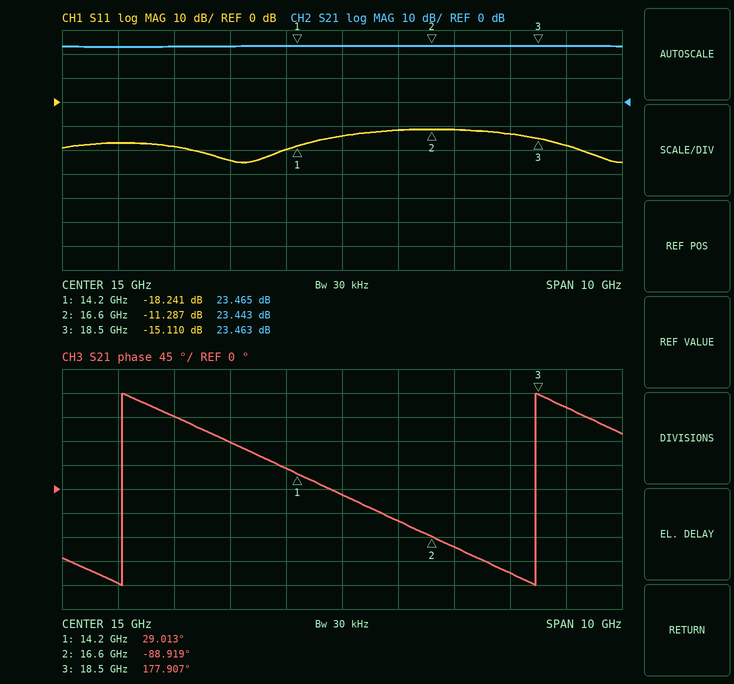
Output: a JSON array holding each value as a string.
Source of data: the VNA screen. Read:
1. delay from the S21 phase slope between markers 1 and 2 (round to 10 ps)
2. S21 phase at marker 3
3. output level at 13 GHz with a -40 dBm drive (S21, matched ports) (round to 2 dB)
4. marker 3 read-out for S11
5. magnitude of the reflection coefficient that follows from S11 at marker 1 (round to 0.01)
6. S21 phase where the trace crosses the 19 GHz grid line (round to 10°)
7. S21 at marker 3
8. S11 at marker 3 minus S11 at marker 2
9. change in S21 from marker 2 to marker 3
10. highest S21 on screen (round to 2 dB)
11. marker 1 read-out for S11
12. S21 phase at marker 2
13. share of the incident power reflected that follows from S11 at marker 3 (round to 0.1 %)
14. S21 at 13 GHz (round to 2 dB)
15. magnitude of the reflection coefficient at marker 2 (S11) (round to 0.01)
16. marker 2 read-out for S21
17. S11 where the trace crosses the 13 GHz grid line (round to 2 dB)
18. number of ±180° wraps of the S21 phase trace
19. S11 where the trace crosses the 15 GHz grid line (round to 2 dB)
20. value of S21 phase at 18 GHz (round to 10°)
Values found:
["140 ps", "177.907°", "-16 dBm", "-15.110 dB", "0.12", "150°", "23.463 dB", "-3.823 dB", "0.020 dB", "24 dB", "-18.241 dB", "-88.919°", "3.1 %", "24 dB", "0.27", "23.443 dB", "-24 dB", "2", "-14 dB", "-160°"]
